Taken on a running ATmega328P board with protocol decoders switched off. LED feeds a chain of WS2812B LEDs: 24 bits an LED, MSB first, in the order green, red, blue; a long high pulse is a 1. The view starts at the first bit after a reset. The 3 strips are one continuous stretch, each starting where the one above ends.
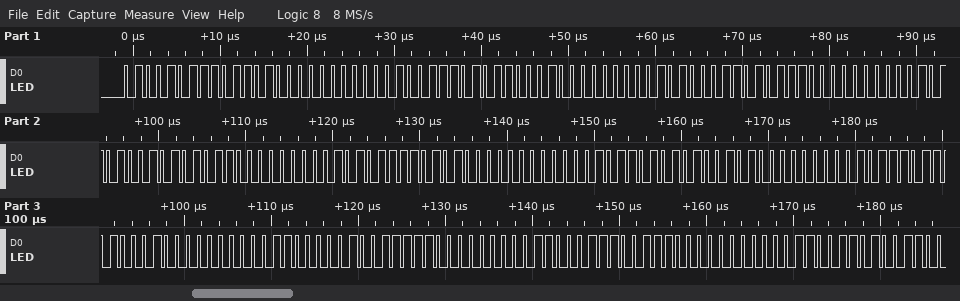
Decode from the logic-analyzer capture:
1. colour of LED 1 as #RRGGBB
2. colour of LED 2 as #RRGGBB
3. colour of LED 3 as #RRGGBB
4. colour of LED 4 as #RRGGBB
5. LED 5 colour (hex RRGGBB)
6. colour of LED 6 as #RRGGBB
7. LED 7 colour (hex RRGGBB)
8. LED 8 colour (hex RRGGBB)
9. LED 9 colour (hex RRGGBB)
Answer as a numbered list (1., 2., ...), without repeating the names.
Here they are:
1. #B44B00
2. #B14E00
3. #AE5100
4. #AB5400
5. #A85700
6. #A55A00
7. #A25D00
8. #9F6000
9. #9C6300
